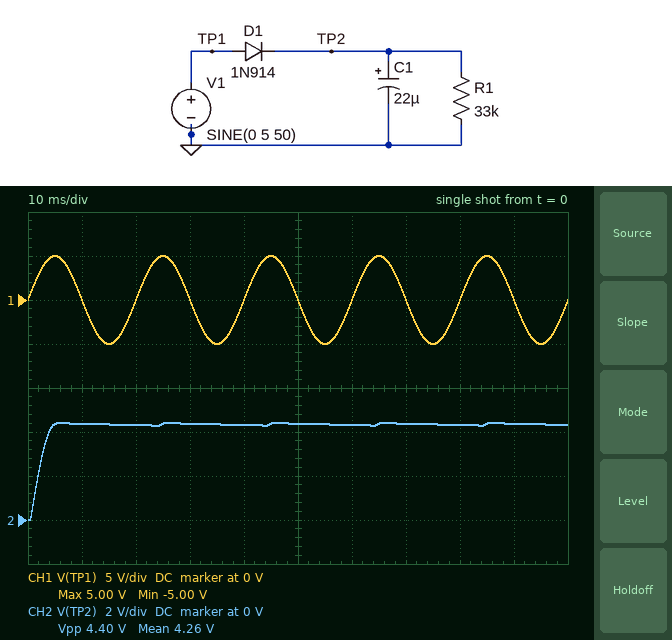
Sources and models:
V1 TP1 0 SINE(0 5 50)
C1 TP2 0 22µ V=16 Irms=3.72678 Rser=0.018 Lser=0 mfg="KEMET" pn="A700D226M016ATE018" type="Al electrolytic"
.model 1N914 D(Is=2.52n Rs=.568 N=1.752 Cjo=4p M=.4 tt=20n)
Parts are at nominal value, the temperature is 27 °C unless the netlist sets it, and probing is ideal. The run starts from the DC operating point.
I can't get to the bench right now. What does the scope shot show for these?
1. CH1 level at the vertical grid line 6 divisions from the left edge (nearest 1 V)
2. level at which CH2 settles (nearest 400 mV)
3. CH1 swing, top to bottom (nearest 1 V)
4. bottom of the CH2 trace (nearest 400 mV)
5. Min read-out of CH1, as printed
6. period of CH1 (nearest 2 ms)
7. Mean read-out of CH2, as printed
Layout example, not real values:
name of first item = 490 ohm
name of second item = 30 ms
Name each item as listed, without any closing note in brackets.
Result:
CH1 level at the vertical grid line 6 divisions from the left edge = 0 V
level at which CH2 settles = 4.4 V
CH1 swing, top to bottom = 10 V
bottom of the CH2 trace = 0 V
Min read-out of CH1, as printed = -5.00 V
period of CH1 = 20 ms
Mean read-out of CH2, as printed = 4.26 V
